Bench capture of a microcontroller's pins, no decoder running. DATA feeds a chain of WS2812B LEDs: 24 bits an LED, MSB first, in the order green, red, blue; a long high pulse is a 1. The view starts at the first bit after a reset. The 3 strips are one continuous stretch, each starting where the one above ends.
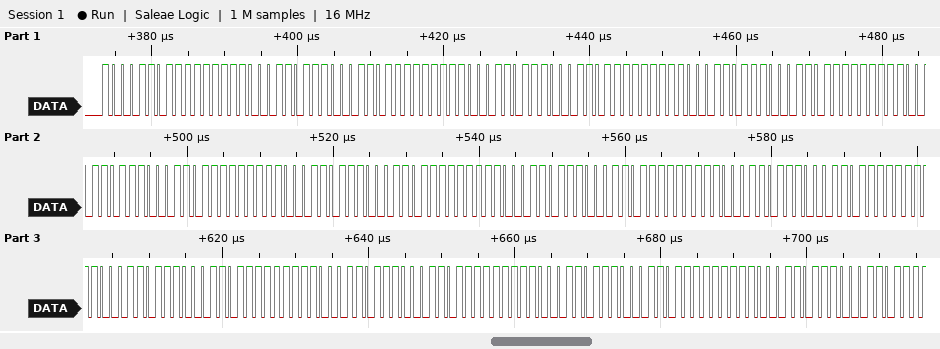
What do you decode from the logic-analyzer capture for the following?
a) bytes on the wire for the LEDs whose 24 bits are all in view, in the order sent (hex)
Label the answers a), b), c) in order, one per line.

a) 8D FF 1B 8D FF 1B 8D FF 1B 8D FF 1B 8D FF 1B 8D FF 1B 8D FF 1B 8D FF 1B 8D FF 1B 8D FF 1B 8D FF 1B
